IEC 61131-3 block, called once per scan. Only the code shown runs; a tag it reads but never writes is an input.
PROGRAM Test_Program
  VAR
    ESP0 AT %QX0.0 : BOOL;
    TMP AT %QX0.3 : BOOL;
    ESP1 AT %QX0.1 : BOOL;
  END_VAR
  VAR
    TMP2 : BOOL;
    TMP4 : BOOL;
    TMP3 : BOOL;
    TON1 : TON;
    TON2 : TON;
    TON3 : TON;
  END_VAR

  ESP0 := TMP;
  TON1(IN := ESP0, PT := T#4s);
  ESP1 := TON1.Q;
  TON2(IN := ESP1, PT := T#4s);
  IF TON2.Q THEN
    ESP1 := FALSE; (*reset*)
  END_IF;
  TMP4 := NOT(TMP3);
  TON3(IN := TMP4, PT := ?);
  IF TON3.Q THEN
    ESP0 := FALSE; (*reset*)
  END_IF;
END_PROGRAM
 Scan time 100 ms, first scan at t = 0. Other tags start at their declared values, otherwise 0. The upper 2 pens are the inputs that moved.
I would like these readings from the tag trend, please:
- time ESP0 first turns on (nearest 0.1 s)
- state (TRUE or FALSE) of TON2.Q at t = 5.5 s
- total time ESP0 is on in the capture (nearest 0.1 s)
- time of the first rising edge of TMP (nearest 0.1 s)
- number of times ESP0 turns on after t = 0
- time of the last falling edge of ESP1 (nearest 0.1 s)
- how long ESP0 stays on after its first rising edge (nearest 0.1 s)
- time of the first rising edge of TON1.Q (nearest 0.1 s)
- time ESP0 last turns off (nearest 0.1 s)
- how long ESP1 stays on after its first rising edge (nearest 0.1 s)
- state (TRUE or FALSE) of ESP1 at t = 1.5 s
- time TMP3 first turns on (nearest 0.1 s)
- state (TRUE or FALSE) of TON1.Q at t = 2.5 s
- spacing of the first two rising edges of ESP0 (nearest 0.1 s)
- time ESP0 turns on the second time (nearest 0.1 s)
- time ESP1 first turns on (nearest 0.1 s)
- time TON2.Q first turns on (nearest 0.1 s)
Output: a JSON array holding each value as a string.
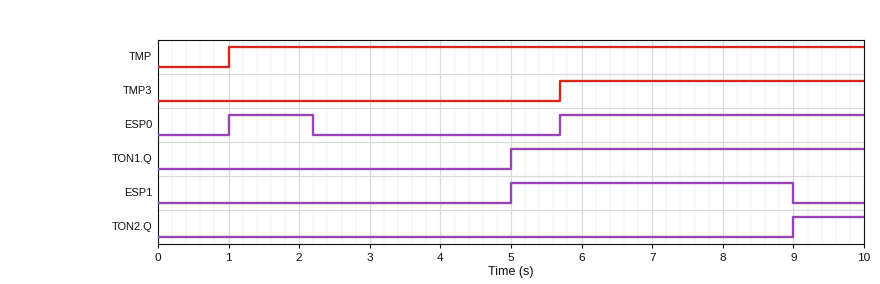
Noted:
["1.0 s", "FALSE", "5.5 s", "1.0 s", "2", "9.0 s", "1.2 s", "5.0 s", "2.2 s", "4.0 s", "FALSE", "5.7 s", "FALSE", "4.7 s", "5.7 s", "5.0 s", "9.0 s"]
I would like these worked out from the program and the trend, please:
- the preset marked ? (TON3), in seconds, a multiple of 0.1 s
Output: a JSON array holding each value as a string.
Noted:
["2.2 s"]
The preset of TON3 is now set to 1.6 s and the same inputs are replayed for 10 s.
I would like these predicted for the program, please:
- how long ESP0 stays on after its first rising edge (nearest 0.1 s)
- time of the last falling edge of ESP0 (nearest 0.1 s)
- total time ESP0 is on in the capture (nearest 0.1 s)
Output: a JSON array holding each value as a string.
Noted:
["0.6 s", "1.6 s", "4.9 s"]
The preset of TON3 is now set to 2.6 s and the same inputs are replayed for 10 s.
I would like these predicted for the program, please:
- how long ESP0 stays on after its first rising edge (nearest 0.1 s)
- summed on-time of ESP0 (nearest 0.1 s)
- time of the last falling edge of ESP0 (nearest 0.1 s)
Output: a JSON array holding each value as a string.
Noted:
["1.6 s", "5.9 s", "2.6 s"]
